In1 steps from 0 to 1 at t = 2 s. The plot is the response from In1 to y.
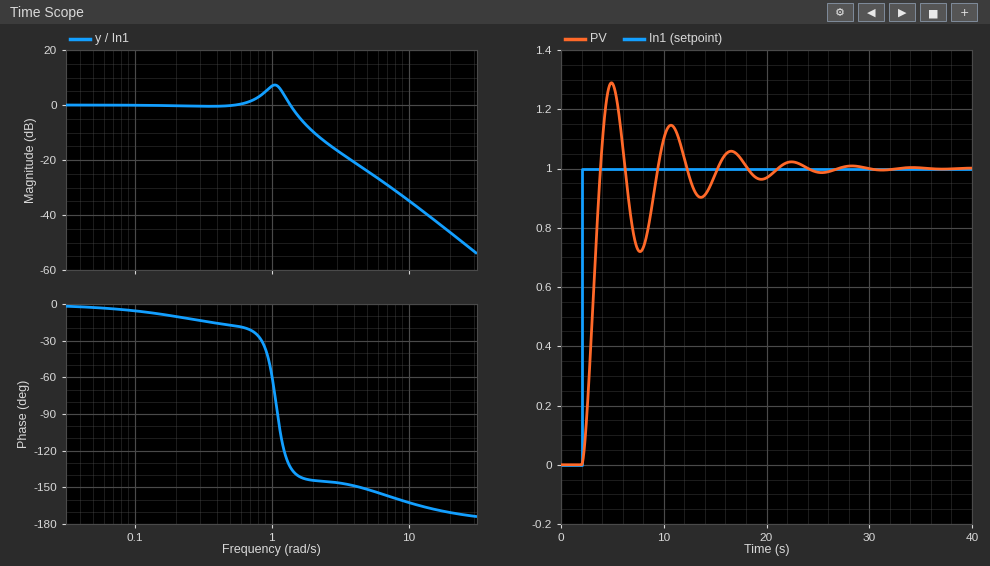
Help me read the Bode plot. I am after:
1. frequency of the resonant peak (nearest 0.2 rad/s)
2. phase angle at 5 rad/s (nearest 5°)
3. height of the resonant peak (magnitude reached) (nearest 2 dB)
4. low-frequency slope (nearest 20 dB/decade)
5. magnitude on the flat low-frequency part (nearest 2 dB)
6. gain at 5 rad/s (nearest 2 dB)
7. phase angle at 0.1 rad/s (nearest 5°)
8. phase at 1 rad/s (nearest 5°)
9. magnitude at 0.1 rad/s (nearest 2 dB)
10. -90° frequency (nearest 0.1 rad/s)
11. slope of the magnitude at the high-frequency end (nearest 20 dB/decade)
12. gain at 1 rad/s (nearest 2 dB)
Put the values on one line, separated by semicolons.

1.0 rad/s; -150°; 8 dB; 0 dB/decade; 0 dB; -24 dB; -5°; -55°; 0 dB; 1.1 rad/s; -40 dB/decade; 6 dB
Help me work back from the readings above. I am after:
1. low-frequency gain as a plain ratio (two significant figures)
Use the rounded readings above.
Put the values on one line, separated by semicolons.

1.0
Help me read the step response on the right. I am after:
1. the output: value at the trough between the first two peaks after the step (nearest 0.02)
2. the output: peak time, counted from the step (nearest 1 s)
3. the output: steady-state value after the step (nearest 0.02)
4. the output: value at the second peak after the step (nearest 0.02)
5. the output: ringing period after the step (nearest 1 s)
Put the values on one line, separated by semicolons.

0.72; 3 s; 1.00; 1.14; 6 s
